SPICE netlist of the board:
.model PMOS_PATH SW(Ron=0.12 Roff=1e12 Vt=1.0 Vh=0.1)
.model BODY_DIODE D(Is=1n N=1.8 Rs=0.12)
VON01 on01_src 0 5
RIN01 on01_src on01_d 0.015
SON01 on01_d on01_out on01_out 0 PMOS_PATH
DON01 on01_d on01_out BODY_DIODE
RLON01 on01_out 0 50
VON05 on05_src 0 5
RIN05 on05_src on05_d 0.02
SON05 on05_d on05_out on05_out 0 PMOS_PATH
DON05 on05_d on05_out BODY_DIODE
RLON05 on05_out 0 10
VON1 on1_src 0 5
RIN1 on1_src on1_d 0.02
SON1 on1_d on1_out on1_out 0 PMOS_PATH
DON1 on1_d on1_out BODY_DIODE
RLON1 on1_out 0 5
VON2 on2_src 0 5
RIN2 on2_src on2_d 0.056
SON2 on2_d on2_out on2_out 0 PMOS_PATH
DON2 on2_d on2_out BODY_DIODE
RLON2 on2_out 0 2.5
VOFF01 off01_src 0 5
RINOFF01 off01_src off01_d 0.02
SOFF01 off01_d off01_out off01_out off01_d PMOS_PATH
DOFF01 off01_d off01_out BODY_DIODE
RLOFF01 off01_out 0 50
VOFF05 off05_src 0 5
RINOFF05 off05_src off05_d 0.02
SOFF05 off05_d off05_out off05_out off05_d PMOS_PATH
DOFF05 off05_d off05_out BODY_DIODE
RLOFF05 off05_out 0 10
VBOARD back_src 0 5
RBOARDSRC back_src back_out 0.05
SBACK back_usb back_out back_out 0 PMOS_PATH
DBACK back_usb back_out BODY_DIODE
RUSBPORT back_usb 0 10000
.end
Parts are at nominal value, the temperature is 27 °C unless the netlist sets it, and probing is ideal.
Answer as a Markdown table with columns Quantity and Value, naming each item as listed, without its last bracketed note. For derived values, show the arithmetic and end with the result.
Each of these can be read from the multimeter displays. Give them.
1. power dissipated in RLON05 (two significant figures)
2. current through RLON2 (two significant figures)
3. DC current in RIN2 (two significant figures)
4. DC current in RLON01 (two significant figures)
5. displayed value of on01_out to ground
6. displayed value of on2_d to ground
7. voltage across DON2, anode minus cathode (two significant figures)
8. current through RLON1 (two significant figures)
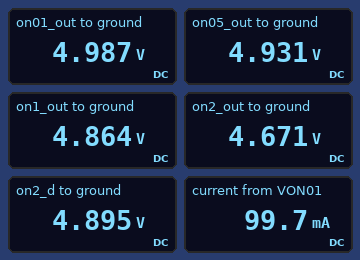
| Quantity | Value |
|---|---|
| power dissipated in RLON05 | (4.931 V)^2 / 10 Ω = 2.4 W |
| current through RLON2 | (4.671 V) / 2.5 Ω = 1.9 A |
| DC current in RIN2 | (5 V - 4.895 V) / 56 mΩ = 1.9 A |
| DC current in RLON01 | (4.987 V) / 50 Ω = 100 mA |
| displayed value of on01_out to ground | 4.987 V |
| displayed value of on2_d to ground | 4.895 V |
| voltage across DON2, anode minus cathode | 4.895 V - 4.671 V = 220 mV |
| current through RLON1 | (4.864 V) / 5 Ω = 970 mA |
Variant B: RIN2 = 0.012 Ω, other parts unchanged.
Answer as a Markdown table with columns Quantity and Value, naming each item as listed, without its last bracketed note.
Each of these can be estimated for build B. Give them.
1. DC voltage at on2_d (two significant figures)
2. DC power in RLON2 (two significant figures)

| Quantity | Value |
|---|---|
| DC voltage at on2_d | 5.0 V |
| DC power in RLON2 | 9.0 W |
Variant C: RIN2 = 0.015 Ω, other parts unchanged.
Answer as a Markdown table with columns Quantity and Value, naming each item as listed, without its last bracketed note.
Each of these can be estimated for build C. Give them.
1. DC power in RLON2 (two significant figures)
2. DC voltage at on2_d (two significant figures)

| Quantity | Value |
|---|---|
| DC power in RLON2 | 9.0 W |
| DC voltage at on2_d | 5.0 V |
